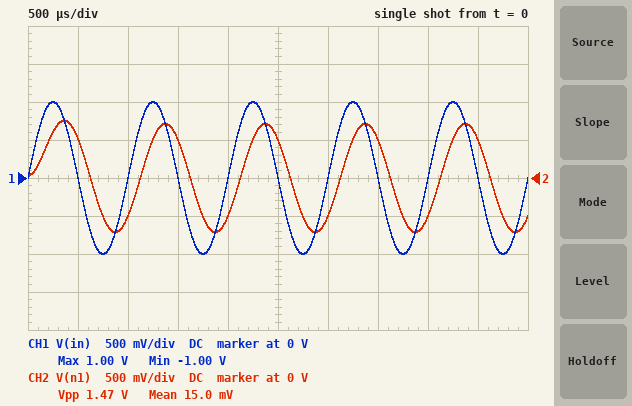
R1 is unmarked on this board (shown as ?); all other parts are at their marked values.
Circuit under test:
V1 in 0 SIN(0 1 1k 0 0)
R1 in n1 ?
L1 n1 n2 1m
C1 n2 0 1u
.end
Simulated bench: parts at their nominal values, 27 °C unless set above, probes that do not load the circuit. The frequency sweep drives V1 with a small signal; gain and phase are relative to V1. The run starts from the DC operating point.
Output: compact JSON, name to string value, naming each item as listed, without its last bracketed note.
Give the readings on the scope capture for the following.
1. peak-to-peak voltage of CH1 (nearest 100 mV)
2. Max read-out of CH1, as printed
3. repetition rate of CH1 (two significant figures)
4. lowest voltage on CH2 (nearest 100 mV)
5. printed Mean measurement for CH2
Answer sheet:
{"peak-to-peak voltage of CH1": "2.0 V", "Max read-out of CH1, as printed": "1.00 V", "repetition rate of CH1": "1.0 kHz", "lowest voltage on CH2": "-700 mV", "printed Mean measurement for CH2": "15.0 mV"}
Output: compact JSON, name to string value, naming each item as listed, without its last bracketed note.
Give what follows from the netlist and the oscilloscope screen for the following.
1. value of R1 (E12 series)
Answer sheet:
{"value of R1": "150 Ω"}
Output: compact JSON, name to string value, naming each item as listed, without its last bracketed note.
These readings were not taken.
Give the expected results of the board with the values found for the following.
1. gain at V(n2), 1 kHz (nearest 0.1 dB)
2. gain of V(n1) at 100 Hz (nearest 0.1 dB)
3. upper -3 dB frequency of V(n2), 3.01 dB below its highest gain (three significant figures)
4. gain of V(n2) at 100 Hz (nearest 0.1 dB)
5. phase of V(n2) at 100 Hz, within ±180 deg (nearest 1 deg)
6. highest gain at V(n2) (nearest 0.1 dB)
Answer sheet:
{"gain at V(n2), 1 kHz": "-2.6 dB", "gain of V(n1) at 100 Hz": "0 dB", "upper -3 dB frequency of V(n2), 3.01 dB below its highest gain": "1.11 kHz", "gain of V(n2) at 100 Hz": "0 dB", "phase of V(n2) at 100 Hz, within ±180 deg": "-5 deg", "highest gain at V(n2)": "0 dB"}
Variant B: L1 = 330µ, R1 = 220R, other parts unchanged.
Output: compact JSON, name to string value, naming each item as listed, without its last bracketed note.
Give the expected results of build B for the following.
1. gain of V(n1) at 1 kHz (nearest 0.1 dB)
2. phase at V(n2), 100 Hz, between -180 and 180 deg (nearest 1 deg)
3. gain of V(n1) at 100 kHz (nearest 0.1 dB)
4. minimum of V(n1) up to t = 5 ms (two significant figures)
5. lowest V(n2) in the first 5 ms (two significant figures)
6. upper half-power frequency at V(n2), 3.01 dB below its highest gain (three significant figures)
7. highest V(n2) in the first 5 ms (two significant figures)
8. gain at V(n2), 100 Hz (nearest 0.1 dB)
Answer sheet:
{"gain of V(n1) at 1 kHz": "-4.7 dB", "phase at V(n2), 100 Hz, between -180 and 180 deg": "-8 deg", "gain of V(n1) at 100 kHz": "-3.3 dB", "minimum of V(n1) up to t = 5 ms": "-580 mV", "lowest V(n2) in the first 5 ms": "-590 mV", "upper half-power frequency at V(n2), 3.01 dB below its highest gain": "728 Hz", "highest V(n2) in the first 5 ms": "670 mV", "gain at V(n2), 100 Hz": "-0.1 dB"}
